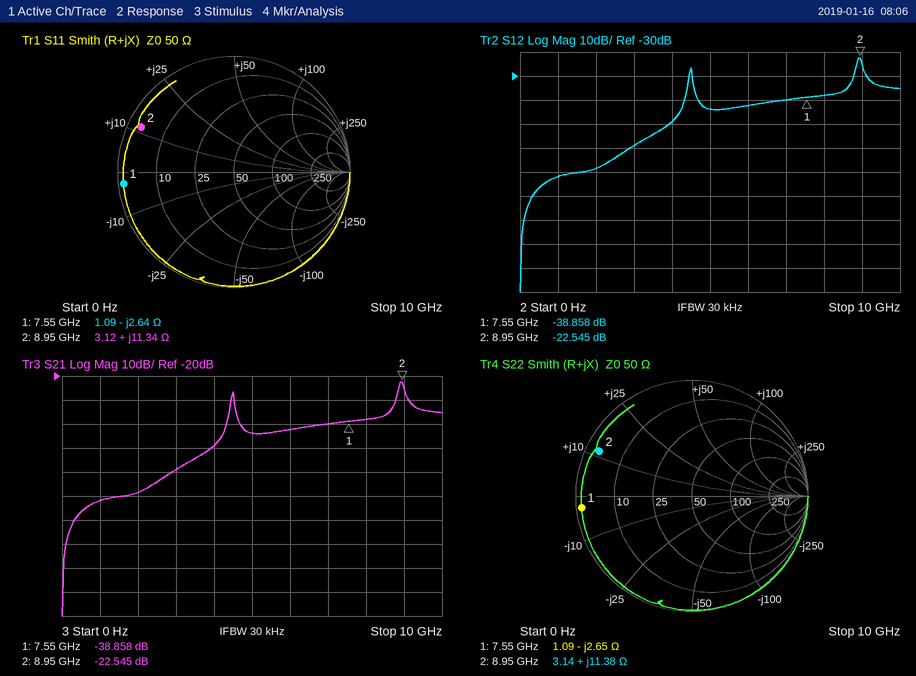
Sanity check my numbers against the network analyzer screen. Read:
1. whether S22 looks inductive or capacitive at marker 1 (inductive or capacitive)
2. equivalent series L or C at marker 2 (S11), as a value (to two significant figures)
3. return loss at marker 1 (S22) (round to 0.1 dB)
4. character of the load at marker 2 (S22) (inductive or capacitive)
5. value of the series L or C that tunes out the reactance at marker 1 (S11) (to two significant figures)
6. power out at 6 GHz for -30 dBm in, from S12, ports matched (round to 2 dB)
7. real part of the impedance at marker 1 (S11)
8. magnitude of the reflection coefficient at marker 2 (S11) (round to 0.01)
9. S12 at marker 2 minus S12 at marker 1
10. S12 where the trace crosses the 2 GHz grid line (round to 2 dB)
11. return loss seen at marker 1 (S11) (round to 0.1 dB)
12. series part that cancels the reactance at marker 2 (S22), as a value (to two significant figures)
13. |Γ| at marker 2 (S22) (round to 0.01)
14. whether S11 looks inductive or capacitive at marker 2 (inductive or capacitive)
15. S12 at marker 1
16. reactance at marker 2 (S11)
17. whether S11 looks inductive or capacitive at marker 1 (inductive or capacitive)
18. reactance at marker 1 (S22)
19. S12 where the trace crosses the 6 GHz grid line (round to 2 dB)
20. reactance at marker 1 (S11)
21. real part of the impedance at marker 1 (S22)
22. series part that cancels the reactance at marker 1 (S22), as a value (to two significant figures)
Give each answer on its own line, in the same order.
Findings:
capacitive
200 pH
0.4 dB
inductive
56 pH
-72 dBm
1.09 Ω
0.89
16.313 dB
-68 dB
0.4 dB
1.6 pF
0.89
inductive
-38.858 dB
+11.34 Ω
capacitive
-2.65 Ω
-42 dB
-2.64 Ω
1.09 Ω
56 pH
